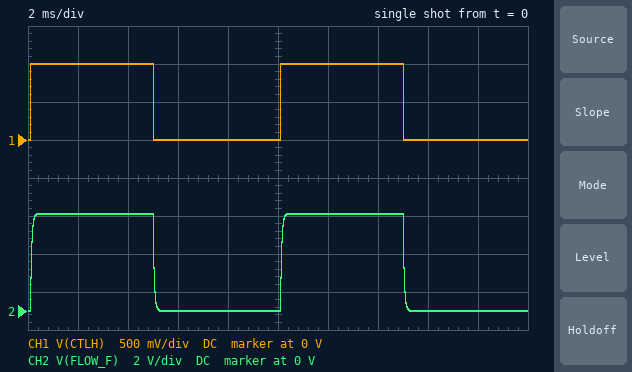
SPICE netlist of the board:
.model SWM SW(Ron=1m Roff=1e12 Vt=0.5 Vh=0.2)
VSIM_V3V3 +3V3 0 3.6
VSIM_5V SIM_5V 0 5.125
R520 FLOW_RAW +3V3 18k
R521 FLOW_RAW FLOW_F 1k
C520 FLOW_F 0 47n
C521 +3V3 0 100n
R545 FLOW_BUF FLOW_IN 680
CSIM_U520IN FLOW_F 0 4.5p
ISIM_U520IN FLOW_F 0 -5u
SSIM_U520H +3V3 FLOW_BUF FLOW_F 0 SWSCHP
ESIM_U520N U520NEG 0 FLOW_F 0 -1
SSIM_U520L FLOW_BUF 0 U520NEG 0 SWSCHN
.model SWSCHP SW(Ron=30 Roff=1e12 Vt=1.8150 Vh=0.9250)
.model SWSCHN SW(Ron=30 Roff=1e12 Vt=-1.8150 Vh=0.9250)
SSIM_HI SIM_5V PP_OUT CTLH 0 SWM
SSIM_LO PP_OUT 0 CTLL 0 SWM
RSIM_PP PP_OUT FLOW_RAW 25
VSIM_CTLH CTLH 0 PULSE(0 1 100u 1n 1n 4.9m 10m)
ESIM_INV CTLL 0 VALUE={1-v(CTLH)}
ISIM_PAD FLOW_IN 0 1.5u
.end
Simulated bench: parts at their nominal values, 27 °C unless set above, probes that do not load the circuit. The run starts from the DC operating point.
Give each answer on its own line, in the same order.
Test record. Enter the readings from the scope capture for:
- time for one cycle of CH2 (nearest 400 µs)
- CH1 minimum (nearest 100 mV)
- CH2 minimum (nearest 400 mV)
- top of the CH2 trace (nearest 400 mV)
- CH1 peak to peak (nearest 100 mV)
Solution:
10.0 ms
0 V
0 V
5.2 V
1.0 V
